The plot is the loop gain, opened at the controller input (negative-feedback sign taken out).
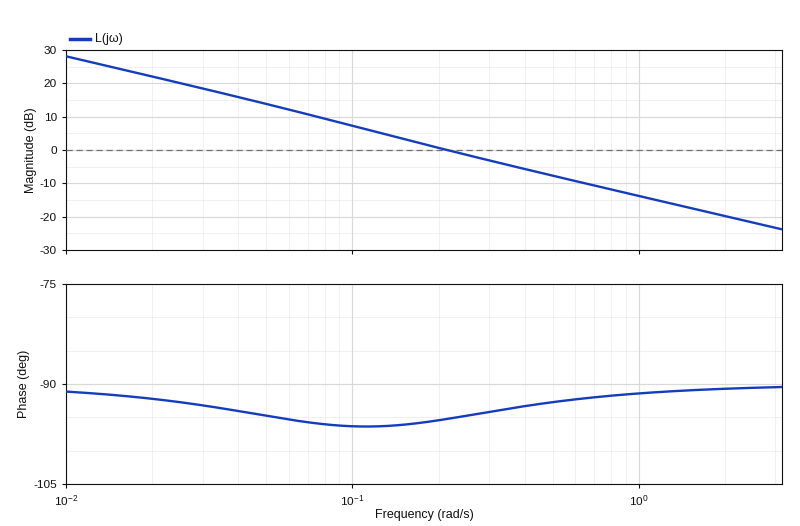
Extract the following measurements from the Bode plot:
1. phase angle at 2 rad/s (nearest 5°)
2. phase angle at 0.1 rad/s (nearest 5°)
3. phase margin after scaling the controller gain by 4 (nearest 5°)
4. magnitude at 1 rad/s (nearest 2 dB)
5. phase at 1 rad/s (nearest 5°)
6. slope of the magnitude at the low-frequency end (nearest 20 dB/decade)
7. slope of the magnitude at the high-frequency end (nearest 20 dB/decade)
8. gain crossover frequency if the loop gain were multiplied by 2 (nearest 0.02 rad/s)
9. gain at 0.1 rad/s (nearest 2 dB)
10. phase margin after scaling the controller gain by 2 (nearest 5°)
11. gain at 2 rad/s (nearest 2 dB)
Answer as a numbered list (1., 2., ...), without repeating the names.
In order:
1. -90°
2. -95°
3. 90°
4. -14 dB
5. -90°
6. -20 dB/decade
7. -20 dB/decade
8. 0.42 rad/s
9. 8 dB
10. 85°
11. -20 dB
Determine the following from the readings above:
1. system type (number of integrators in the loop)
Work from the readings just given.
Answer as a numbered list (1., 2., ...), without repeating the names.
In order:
1. 1
